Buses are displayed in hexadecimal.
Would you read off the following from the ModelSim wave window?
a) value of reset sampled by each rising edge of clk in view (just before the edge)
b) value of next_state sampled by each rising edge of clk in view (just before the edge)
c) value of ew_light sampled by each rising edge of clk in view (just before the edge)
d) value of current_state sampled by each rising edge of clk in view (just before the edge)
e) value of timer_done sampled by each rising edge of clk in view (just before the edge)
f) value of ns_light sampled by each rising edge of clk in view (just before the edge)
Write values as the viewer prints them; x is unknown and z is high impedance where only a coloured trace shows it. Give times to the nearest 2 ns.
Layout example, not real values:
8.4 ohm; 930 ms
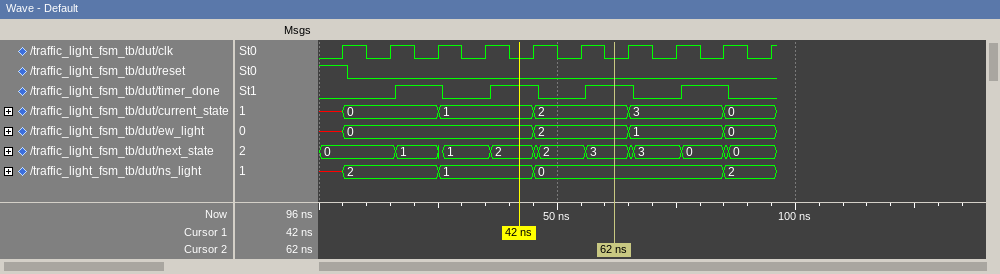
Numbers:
1 0 0 0 0 0 0 0 0 0; 0, 0, 1, 1, 2, 2, 3, 3, 0, 0; x, 0, 0, 0, 0, 2, 2, 1, 1, 0; x, 0, 0, 1, 1, 2, 2, 3, 3, 0; 0 0 1 0 1 0 1 0 1 0; x, 2, 2, 1, 1, 0, 0, 0, 0, 2
